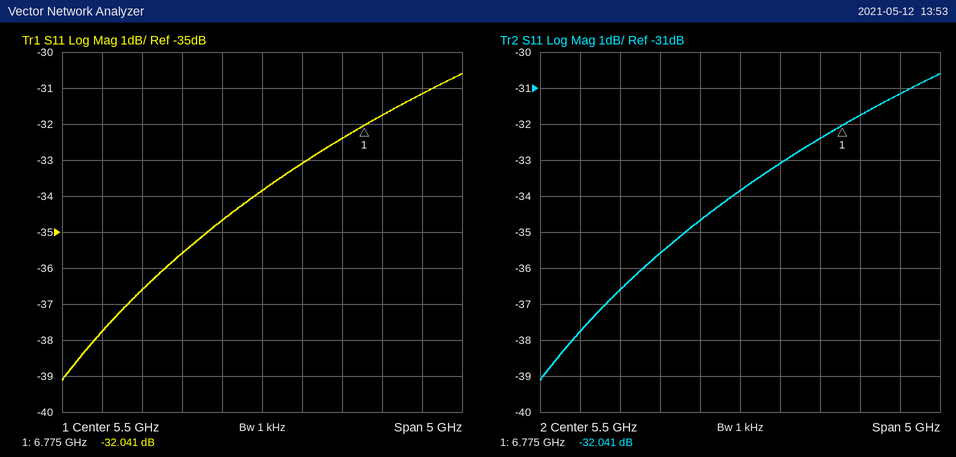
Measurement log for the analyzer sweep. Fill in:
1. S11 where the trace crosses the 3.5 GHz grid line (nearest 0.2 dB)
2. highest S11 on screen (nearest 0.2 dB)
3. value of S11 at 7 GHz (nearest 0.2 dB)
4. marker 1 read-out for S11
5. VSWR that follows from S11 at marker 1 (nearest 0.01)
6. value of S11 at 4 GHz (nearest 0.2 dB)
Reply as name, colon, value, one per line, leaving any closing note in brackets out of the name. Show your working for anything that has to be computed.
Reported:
S11 where the trace crosses the 3.5 GHz grid line: -37.8 dB
highest S11 on screen: -30.6 dB
value of S11 at 7 GHz: -31.8 dB
marker 1 read-out for S11: -32.041 dB
VSWR that follows from S11 at marker 1: (1 + 0.0250)/(1 − 0.0250) ≈ 1.05
value of S11 at 4 GHz: -36.6 dB
